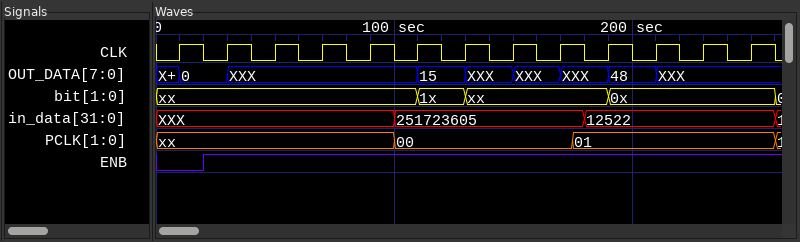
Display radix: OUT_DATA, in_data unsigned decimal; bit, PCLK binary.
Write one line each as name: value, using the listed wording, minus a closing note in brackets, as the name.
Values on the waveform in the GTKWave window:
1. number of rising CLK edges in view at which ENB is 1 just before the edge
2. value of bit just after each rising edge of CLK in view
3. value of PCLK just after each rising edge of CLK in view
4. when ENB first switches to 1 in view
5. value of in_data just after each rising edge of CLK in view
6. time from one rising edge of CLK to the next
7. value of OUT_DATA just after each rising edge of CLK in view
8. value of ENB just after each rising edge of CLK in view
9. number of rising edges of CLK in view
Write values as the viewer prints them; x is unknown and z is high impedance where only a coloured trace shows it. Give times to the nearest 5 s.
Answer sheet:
number of rising CLK edges in view at which ENB is 1 just before the edge: 12
value of bit just after each rising edge of CLK in view: xx, xx, xx, xx, xx, 1x, xx, xx, xx, 0x, 0x, 0x, 0x
value of PCLK just after each rising edge of CLK in view: xx, xx, xx, xx, xx, 00, 00, 00, 00, 01, 01, 01, 01
when ENB first switches to 1 in view: 20 s
value of in_data just after each rising edge of CLK in view: XXX, XXX, XXX, XXX, XXX, 251723605, 251723605, 251723605, 251723605, 12522, 12522, 12522, 12522
time from one rising edge of CLK to the next: 20 s
value of OUT_DATA just after each rising edge of CLK in view: 0, XXX, XXX, XXX, XXX, 15, XXX, XXX, XXX, 48, XXX, XXX, XXX
value of ENB just after each rising edge of CLK in view: 0 1 1 1 1 1 1 1 1 1 1 1 1
number of rising edges of CLK in view: 13
